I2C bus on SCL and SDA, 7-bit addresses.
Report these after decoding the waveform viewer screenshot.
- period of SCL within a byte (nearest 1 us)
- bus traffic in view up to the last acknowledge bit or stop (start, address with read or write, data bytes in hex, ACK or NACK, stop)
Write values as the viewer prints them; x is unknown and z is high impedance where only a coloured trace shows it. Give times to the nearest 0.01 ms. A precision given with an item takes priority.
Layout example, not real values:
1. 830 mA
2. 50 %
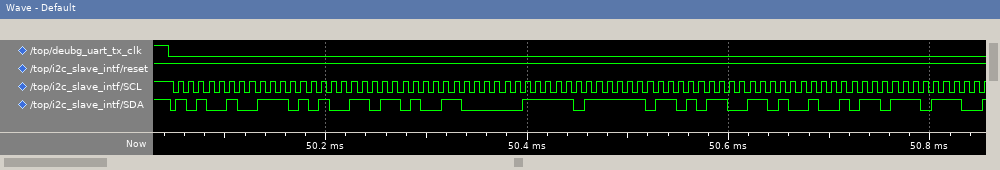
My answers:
1. 10 us
2. start, address 52 write NACK, D4 NACK, B4 NACK, 81 NACK, EF NACK, B5 NACK, 34 NACK, 2D NACK
